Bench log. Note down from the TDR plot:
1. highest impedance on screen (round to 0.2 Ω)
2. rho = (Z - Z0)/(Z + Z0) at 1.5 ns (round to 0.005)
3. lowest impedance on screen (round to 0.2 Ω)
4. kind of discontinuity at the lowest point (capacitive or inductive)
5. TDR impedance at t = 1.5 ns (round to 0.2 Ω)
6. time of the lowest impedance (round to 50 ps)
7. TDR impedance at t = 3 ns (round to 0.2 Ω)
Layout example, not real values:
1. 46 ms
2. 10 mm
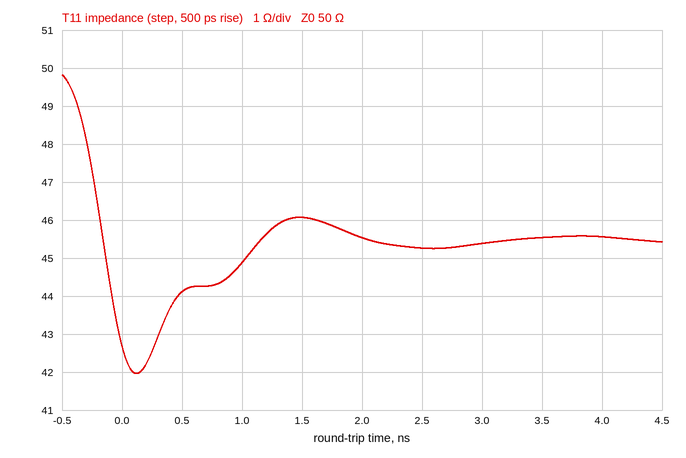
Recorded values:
1. 49.8 Ω
2. -0.040
3. 42.0 Ω
4. capacitive
5. 46.0 Ω
6. 100 ps
7. 45.4 Ω
